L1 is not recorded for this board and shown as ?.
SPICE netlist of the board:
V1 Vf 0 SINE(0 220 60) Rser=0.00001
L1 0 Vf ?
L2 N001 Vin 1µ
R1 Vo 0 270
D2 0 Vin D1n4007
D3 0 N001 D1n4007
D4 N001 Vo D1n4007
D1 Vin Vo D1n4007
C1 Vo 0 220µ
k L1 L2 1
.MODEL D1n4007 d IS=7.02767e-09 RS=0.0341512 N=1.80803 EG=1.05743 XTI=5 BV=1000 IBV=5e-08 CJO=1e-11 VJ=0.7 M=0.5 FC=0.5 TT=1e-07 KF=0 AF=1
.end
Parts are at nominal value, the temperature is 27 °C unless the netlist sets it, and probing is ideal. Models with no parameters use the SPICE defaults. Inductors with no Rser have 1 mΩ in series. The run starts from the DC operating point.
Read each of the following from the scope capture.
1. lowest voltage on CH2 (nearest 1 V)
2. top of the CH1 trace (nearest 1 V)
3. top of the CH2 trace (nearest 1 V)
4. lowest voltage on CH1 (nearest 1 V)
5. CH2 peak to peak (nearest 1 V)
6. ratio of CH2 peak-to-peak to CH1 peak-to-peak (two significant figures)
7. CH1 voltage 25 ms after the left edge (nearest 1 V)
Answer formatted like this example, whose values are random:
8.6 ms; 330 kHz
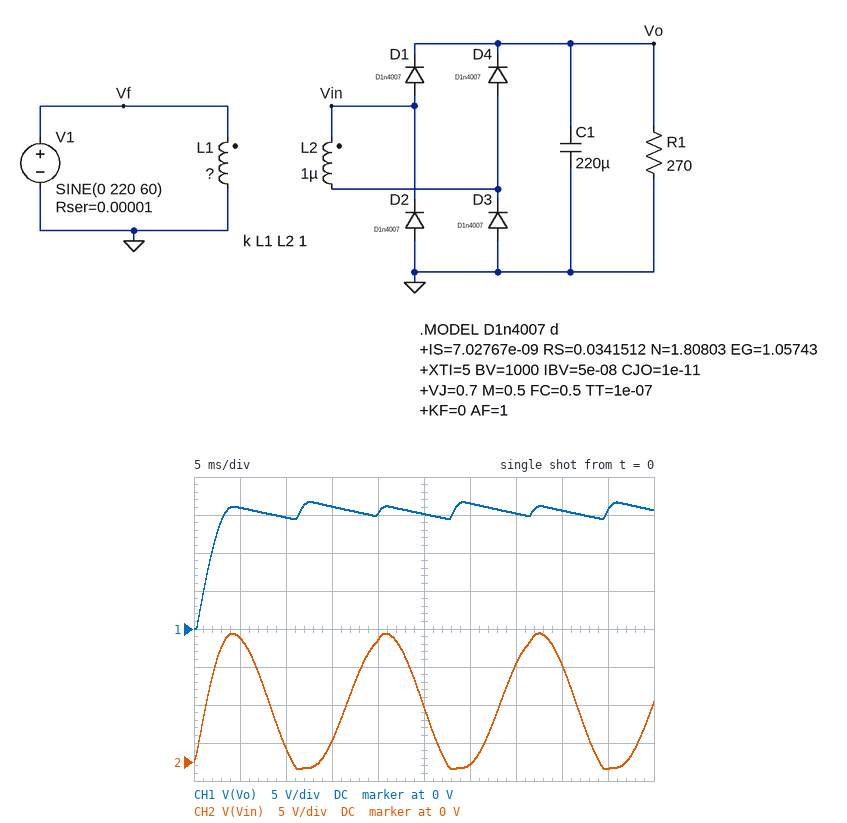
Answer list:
-1 V; 17 V; 17 V; 0 V; 18 V; 1.1; 15 V
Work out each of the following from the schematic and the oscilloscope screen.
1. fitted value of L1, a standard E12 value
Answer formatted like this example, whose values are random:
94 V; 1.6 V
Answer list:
150 µH
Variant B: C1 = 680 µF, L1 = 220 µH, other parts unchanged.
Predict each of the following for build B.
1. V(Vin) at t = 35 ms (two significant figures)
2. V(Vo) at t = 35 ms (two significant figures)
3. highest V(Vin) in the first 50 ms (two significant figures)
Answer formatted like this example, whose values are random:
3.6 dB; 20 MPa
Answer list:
11 V; 13 V; 14 V
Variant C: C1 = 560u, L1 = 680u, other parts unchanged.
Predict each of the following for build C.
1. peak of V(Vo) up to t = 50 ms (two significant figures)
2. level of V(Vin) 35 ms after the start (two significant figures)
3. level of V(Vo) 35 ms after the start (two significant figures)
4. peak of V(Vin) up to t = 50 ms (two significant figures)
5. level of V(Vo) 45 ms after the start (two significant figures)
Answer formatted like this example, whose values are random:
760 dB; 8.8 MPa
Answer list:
6.9 V; 5.8 V; 6.7 V; 7.6 V; 6.6 V
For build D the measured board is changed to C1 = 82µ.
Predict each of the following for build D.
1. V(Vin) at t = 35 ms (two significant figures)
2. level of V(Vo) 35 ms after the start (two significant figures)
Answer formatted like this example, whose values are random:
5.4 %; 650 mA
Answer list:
12 V; 13 V
